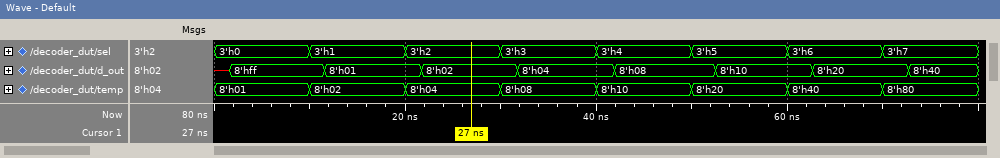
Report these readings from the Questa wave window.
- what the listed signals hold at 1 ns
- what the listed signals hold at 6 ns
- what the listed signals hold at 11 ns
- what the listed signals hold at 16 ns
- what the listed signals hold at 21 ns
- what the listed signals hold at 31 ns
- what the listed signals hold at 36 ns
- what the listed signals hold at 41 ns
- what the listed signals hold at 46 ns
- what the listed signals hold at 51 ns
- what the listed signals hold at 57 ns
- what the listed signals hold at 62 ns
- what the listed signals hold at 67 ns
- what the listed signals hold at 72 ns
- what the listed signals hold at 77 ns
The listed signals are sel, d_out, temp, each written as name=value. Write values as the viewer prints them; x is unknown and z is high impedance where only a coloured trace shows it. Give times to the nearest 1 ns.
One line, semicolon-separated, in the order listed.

sel=3'h0, d_out=x, temp=8'h01; sel=3'h0, d_out=8'hff, temp=8'h01; sel=3'h1, d_out=8'hff, temp=8'h02; sel=3'h1, d_out=8'h01, temp=8'h02; sel=3'h2, d_out=8'h01, temp=8'h04; sel=3'h3, d_out=8'h02, temp=8'h08; sel=3'h3, d_out=8'h04, temp=8'h08; sel=3'h4, d_out=8'h04, temp=8'h10; sel=3'h4, d_out=8'h08, temp=8'h10; sel=3'h5, d_out=8'h08, temp=8'h20; sel=3'h5, d_out=8'h10, temp=8'h20; sel=3'h6, d_out=8'h10, temp=8'h40; sel=3'h6, d_out=8'h20, temp=8'h40; sel=3'h7, d_out=8'h20, temp=8'h80; sel=3'h7, d_out=8'h40, temp=8'h80
